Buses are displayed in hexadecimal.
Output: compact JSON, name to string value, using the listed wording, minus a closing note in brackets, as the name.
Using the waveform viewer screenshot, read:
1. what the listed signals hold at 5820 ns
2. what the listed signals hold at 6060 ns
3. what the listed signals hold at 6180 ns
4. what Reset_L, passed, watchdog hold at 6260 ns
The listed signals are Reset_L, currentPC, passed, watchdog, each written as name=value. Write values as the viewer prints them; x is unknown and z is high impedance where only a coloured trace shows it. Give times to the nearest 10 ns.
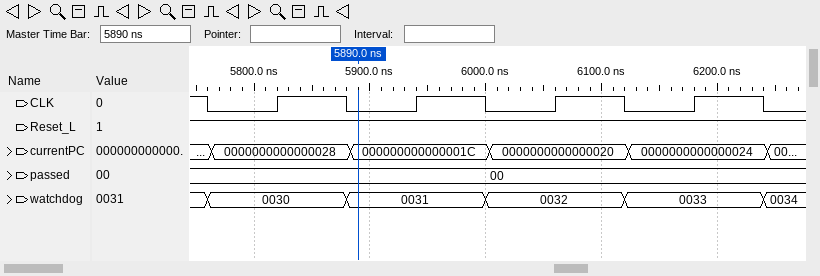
{"what the listed signals hold at 5820 ns": "Reset_L=1, currentPC=0000000000000028, passed=00, watchdog=0030", "what the listed signals hold at 6060 ns": "Reset_L=1, currentPC=0000000000000020, passed=00, watchdog=0032", "what the listed signals hold at 6180 ns": "Reset_L=1, currentPC=0000000000000024, passed=00, watchdog=0033", "what Reset_L, passed, watchdog hold at 6260 ns": "Reset_L=1, passed=00, watchdog=0034"}
